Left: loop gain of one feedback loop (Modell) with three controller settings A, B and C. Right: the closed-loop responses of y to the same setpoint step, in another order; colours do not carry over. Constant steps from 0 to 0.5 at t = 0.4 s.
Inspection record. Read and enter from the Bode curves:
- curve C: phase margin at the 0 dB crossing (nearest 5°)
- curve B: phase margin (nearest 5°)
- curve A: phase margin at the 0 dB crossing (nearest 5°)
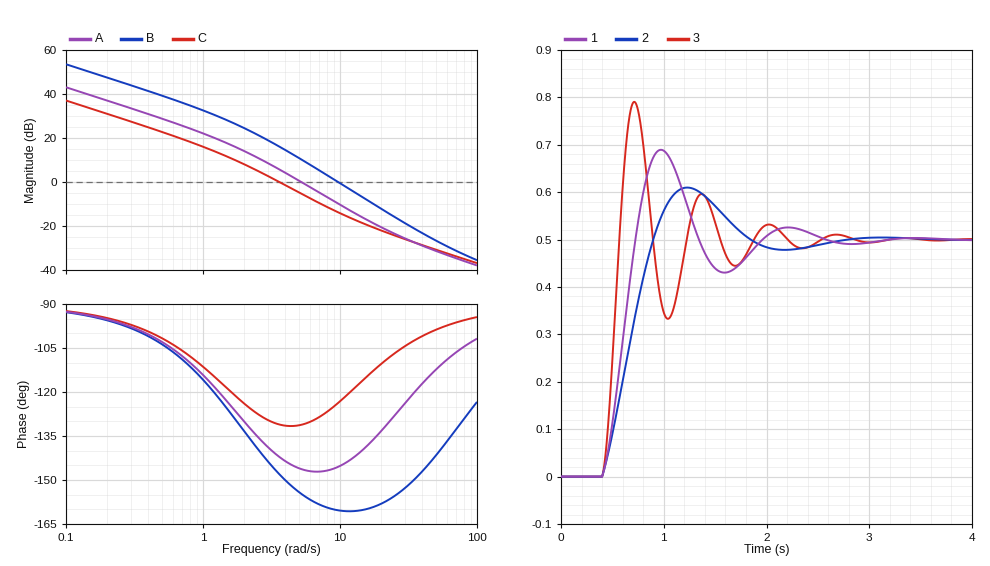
50°
20°
35°
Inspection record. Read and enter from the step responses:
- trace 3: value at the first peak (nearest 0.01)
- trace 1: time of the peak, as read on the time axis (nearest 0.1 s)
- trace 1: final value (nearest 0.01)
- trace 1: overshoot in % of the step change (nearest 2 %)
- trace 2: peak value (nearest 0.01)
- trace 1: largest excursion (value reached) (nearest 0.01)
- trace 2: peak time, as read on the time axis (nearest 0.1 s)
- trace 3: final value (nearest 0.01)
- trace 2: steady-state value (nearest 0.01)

0.79
1.0 s
0.50
38 %
0.61
0.69
1.2 s
0.50
0.50
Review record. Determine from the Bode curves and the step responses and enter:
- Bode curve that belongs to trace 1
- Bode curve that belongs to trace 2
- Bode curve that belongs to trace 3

A
C
B
